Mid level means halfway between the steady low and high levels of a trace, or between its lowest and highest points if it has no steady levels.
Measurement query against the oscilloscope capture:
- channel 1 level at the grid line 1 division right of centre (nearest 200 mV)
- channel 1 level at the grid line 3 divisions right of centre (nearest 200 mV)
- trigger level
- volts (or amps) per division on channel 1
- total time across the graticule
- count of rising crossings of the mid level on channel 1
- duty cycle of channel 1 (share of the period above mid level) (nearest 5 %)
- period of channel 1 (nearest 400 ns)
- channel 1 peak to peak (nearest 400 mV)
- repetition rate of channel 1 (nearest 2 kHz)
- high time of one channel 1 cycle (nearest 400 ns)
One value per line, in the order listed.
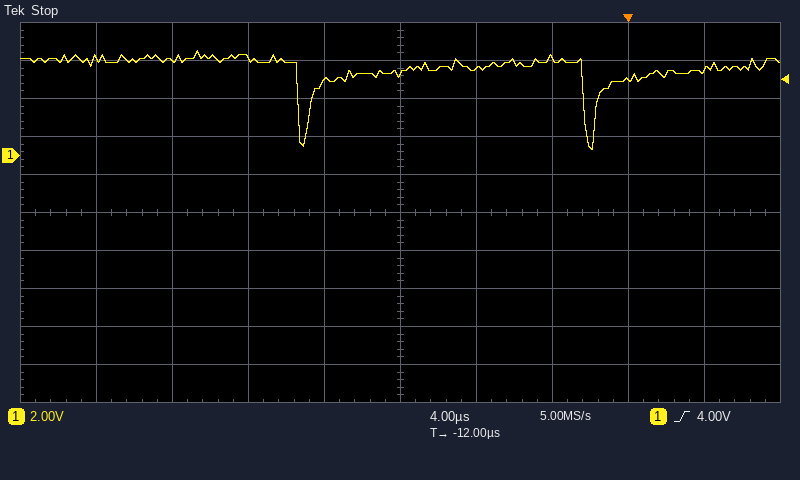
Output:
4.6 V
4.0 V
4.00 V
2 V
40 µs
2
95 %
15.2 µs
5.2 V
66 kHz
14.4 µs
